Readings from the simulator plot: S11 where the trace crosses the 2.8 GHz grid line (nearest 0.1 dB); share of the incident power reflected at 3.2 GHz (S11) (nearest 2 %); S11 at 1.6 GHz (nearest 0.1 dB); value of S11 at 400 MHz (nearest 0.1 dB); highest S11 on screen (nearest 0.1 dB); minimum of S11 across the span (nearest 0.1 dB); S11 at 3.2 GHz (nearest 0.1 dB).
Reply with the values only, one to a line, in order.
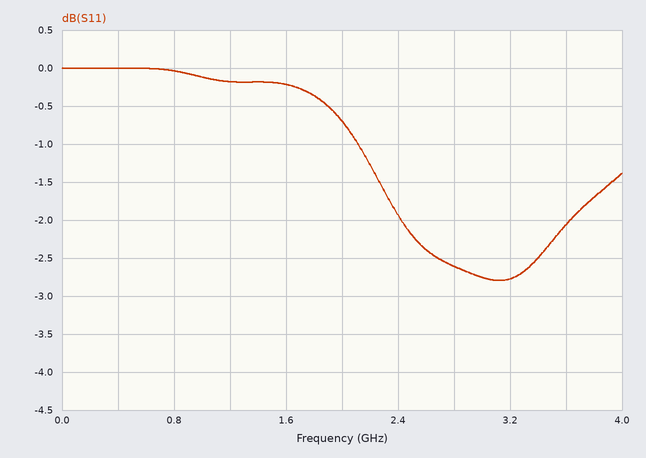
-2.6 dB
52 %
-0.2 dB
0.0 dB
0.0 dB
-2.8 dB
-2.8 dB
